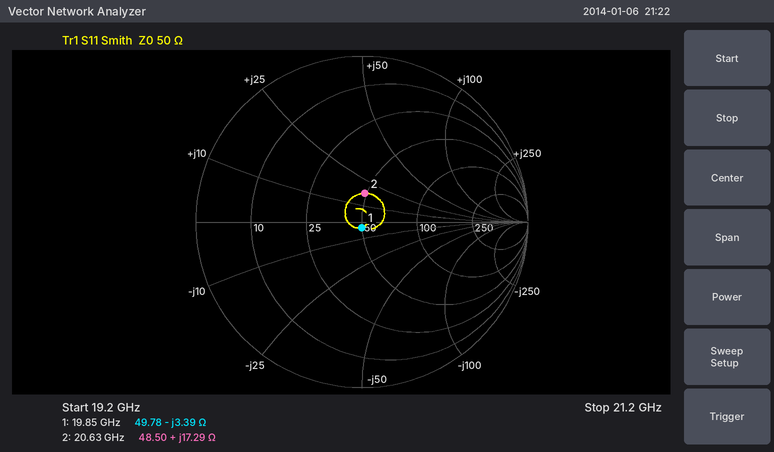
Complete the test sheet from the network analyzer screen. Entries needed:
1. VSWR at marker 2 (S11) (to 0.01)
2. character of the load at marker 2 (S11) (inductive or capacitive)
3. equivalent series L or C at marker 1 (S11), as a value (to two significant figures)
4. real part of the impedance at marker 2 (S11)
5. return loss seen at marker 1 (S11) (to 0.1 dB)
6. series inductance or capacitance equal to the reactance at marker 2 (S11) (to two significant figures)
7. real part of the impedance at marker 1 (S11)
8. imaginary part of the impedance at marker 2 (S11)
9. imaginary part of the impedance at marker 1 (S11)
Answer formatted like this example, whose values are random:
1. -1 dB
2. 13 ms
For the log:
1. 1.42
2. inductive
3. 2.4 pF
4. 48.50 Ω
5. 29.4 dB
6. 130 pH
7. 49.78 Ω
8. +17.29 Ω
9. -3.39 Ω
